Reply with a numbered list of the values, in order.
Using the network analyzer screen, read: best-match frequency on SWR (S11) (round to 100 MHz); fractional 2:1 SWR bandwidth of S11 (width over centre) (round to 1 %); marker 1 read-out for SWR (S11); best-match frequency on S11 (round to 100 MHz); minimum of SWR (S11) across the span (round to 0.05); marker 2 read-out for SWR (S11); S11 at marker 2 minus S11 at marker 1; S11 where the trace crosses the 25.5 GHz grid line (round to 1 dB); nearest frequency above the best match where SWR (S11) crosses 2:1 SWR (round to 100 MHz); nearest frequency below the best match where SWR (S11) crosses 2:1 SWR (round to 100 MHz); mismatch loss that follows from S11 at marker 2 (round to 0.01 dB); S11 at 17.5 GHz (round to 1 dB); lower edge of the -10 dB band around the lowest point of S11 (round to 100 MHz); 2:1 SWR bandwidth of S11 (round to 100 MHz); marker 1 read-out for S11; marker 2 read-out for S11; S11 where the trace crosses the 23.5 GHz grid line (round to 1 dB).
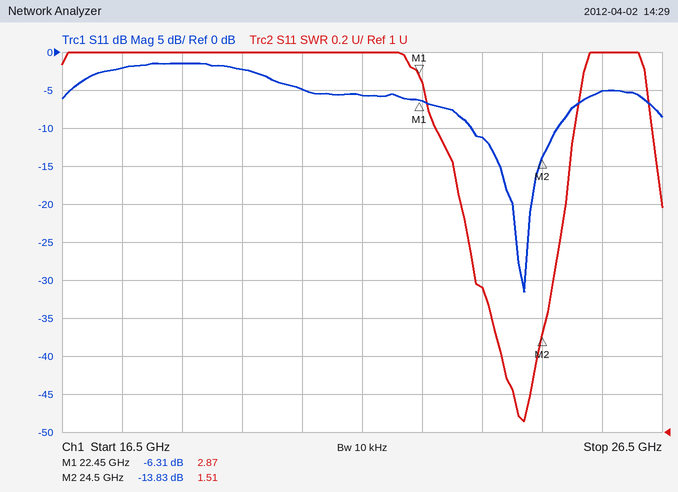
1. 24.2 GHz
2. 6 %
3. 2.87
4. 24.2 GHz
5. 1.05
6. 1.51
7. -7.52 dB
8. -5 dB
9. 24.8 GHz
10. 23.3 GHz
11. 0.18 dB
12. -2 dB
13. 23.3 GHz
14. 1.5 GHz
15. -6.31 dB
16. -13.83 dB
17. -11 dB
